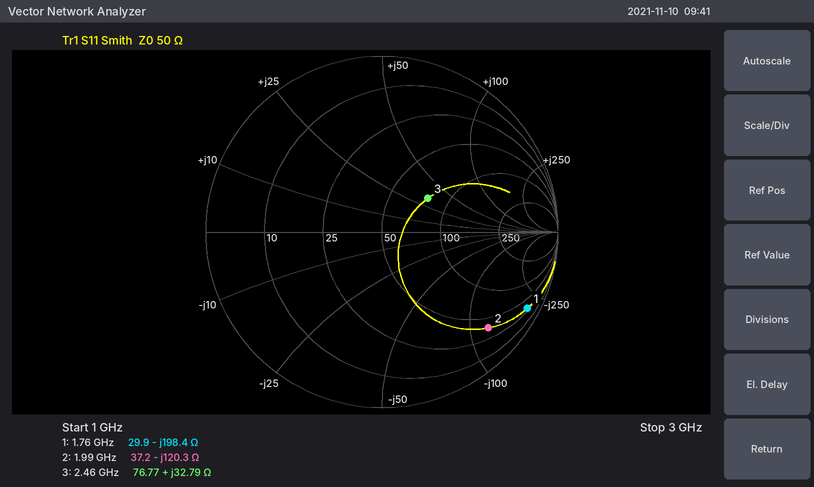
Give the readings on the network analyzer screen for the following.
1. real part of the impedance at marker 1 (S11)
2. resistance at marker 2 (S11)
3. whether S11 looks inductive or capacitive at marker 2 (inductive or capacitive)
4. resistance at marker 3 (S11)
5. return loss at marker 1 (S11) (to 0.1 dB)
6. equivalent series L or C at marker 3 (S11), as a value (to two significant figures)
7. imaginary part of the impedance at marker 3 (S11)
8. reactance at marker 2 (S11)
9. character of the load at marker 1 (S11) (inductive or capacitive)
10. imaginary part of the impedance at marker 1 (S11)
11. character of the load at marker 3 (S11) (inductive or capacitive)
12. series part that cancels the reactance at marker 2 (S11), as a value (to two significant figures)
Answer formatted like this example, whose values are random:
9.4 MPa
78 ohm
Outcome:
29.9 Ω
37.2 Ω
capacitive
76.77 Ω
0.6 dB
2.1 nH
+32.79 Ω
-120.3 Ω
capacitive
-198.4 Ω
inductive
9.6 nH
